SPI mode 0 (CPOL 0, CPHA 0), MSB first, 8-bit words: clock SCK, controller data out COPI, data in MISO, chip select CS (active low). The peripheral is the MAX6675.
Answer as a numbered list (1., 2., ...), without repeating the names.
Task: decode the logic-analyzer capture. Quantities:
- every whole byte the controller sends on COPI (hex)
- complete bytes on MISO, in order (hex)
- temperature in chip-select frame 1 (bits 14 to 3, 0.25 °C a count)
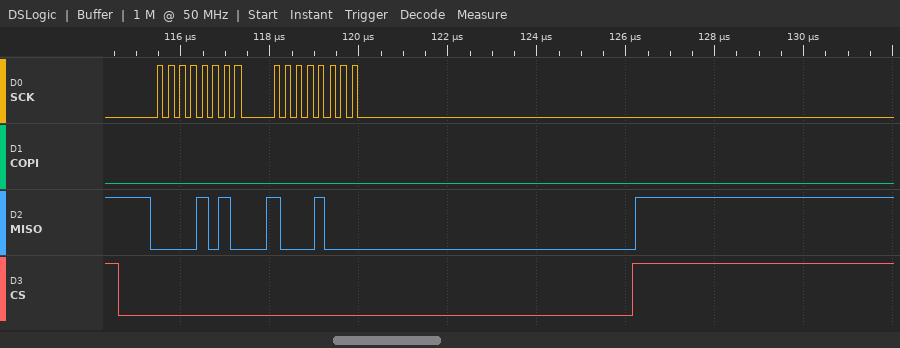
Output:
1. 0x00 0x00
2. 0x0A 0x88
3. 84.25 °C
